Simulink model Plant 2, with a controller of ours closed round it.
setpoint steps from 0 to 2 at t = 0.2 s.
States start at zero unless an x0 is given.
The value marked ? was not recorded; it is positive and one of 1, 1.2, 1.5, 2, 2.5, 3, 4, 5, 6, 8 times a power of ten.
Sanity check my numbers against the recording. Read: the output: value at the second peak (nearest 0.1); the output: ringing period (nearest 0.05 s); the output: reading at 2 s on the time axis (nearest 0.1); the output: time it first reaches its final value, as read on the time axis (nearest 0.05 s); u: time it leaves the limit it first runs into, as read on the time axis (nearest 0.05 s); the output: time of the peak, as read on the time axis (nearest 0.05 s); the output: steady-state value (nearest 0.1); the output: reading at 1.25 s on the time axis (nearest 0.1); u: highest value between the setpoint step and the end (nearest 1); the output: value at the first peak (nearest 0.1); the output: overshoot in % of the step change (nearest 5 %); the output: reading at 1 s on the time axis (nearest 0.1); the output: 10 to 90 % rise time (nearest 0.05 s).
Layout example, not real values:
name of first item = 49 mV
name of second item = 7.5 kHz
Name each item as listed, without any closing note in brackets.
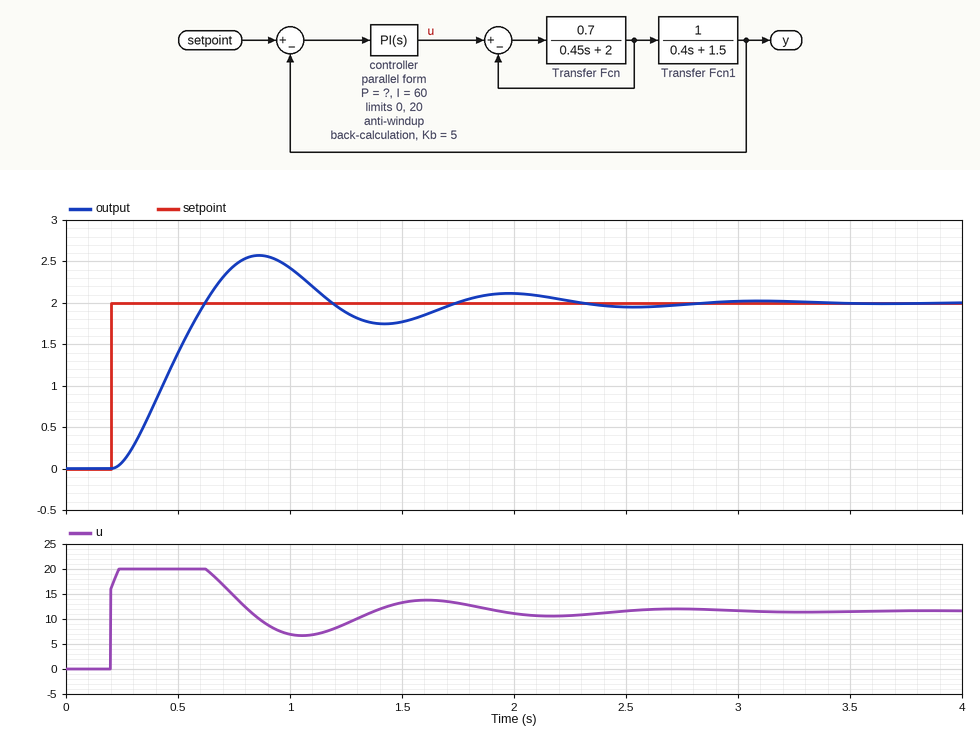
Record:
the output: value at the second peak = 2.1
the output: ringing period = 1.10 s
the output: reading at 2 s on the time axis = 2.1
the output: time it first reaches its final value, as read on the time axis = 0.60 s
u: time it leaves the limit it first runs into, as read on the time axis = 0.65 s
the output: time of the peak, as read on the time axis = 0.85 s
the output: steady-state value = 2.0
the output: reading at 1.25 s on the time axis = 1.9
u: highest value between the setpoint step and the end = 20
the output: value at the first peak = 2.6
the output: overshoot in % of the step change = 30 %
the output: reading at 1 s on the time axis = 2.4
the output: 10 to 90 % rise time = 0.30 s
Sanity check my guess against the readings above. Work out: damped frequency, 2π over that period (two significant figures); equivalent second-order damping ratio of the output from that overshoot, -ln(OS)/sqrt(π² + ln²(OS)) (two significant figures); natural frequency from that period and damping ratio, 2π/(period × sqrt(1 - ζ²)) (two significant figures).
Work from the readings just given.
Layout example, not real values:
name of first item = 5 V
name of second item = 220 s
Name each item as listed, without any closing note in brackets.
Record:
damped frequency, 2π over that period = 5.7 rad/s
equivalent second-order damping ratio of the output from that overshoot, -ln(OS)/sqrt(π² + ln²(OS)) = 0.36
natural frequency from that period and damping ratio, 2π/(period × sqrt(1 - ζ²)) = 6.1 rad/s
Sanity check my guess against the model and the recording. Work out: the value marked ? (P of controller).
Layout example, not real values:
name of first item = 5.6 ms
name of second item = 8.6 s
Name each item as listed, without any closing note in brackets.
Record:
the value marked ? = 8
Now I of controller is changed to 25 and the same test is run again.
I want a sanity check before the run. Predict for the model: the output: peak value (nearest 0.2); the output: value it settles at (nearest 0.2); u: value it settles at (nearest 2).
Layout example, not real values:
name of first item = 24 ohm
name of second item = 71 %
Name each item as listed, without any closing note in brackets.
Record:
the output: peak value = 2.2
the output: value it settles at = 2.0
u: value it settles at = 12
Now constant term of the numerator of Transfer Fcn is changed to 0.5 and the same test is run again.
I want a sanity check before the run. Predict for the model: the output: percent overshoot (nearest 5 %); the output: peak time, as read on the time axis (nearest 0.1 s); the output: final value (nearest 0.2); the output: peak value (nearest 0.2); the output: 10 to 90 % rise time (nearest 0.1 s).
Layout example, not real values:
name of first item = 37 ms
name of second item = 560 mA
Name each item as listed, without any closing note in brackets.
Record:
the output: percent overshoot = 15 %
the output: peak time, as read on the time axis = 1.1 s
the output: final value = 2.0
the output: peak value = 2.4
the output: 10 to 90 % rise time = 0.4 s
